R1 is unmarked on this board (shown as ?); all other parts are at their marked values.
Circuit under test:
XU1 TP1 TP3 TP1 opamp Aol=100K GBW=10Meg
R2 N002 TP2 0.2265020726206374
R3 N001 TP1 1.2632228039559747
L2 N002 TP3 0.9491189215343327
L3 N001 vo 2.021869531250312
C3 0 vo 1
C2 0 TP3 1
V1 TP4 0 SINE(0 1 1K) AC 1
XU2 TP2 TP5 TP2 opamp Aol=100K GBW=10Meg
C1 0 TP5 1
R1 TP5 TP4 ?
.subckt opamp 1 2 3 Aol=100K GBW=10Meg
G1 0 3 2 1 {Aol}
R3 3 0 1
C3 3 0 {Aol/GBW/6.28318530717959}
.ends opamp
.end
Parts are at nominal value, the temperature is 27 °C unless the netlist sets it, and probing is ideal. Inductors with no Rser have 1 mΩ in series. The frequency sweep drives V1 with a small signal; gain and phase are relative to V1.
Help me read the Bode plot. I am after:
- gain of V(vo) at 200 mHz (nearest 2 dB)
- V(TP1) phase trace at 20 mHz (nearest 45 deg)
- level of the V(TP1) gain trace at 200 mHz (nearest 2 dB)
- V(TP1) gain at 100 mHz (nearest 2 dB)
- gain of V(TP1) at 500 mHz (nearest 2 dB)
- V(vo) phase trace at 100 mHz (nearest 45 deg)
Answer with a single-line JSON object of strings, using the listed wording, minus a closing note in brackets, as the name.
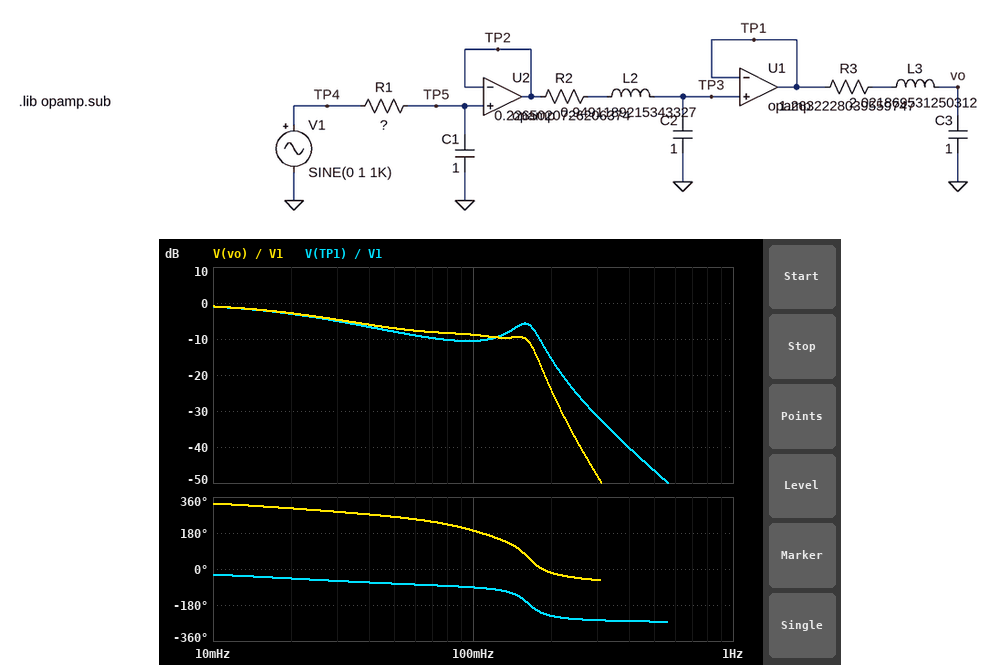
{"gain of V(vo) at 200 mHz": "-24 dB", "V(TP1) phase trace at 20 mHz": "-45 deg", "level of the V(TP1) gain trace at 200 mHz": "-16 dB", "V(TP1) gain at 100 mHz": "-10 dB", "gain of V(TP1) at 500 mHz": "-46 dB", "V(vo) phase trace at 100 mHz": "180 deg"}
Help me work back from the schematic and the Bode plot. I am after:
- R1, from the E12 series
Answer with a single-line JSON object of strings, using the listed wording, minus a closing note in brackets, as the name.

{"R1, from the E12 series": "8.2 Ω"}
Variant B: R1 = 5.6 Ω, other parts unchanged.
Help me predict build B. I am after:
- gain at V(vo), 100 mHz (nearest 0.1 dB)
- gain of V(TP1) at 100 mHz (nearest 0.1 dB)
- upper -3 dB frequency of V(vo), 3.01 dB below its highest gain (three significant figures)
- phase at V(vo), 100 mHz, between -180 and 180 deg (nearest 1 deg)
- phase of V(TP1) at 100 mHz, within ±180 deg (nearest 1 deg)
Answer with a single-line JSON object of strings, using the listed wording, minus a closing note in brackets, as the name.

{"gain at V(vo), 100 mHz": "-5.7 dB", "gain of V(TP1) at 100 mHz": "-7.4 dB", "upper -3 dB frequency of V(vo), 3.01 dB below its highest gain": "34.0 mHz", "phase at V(vo), 100 mHz, between -180 and 180 deg": "-163 deg", "phase of V(TP1) at 100 mHz, within ±180 deg": "-87 deg"}
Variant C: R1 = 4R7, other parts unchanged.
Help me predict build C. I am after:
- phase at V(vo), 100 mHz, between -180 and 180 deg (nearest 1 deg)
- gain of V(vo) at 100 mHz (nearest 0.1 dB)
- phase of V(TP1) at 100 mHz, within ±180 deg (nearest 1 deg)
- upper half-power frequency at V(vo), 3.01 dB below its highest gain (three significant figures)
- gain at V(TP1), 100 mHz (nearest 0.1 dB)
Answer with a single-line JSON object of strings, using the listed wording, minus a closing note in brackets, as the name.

{"phase at V(vo), 100 mHz, between -180 and 180 deg": "-160 deg", "gain of V(vo) at 100 mHz": "-4.3 dB", "phase of V(TP1) at 100 mHz, within ±180 deg": "-84 deg", "upper half-power frequency at V(vo), 3.01 dB below its highest gain": "46.1 mHz", "gain at V(TP1), 100 mHz": "-6.0 dB"}
